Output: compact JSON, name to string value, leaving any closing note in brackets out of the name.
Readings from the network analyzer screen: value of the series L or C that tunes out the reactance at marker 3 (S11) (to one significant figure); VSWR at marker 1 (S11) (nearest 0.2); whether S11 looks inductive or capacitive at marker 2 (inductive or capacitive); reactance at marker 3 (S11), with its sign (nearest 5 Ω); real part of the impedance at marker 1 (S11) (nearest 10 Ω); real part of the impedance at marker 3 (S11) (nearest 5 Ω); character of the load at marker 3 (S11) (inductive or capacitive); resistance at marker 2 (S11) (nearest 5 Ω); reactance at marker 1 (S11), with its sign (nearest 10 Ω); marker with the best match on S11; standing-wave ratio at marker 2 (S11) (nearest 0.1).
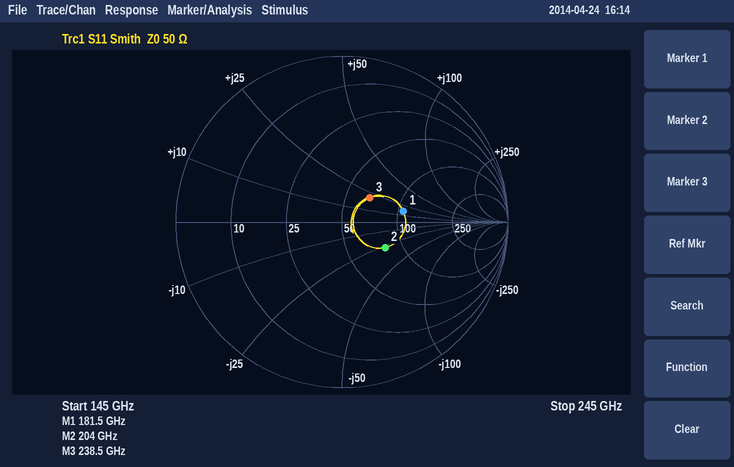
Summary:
{"value of the series L or C that tunes out the reactance at marker 3 (S11)": "30 fF", "VSWR at marker 1 (S11)": "2.2", "whether S11 looks inductive or capacitive at marker 2": "capacitive", "reactance at marker 3 (S11), with its sign": "+20 Ω", "real part of the impedance at marker 1 (S11)": "110 Ω", "real part of the impedance at marker 3 (S11)": "65 Ω", "character of the load at marker 3 (S11)": "inductive", "resistance at marker 2 (S11)": "80 Ω", "reactance at marker 1 (S11), with its sign": "+20 Ω", "marker with the best match on S11": "marker 3", "standing-wave ratio at marker 2 (S11)": "1.9"}
